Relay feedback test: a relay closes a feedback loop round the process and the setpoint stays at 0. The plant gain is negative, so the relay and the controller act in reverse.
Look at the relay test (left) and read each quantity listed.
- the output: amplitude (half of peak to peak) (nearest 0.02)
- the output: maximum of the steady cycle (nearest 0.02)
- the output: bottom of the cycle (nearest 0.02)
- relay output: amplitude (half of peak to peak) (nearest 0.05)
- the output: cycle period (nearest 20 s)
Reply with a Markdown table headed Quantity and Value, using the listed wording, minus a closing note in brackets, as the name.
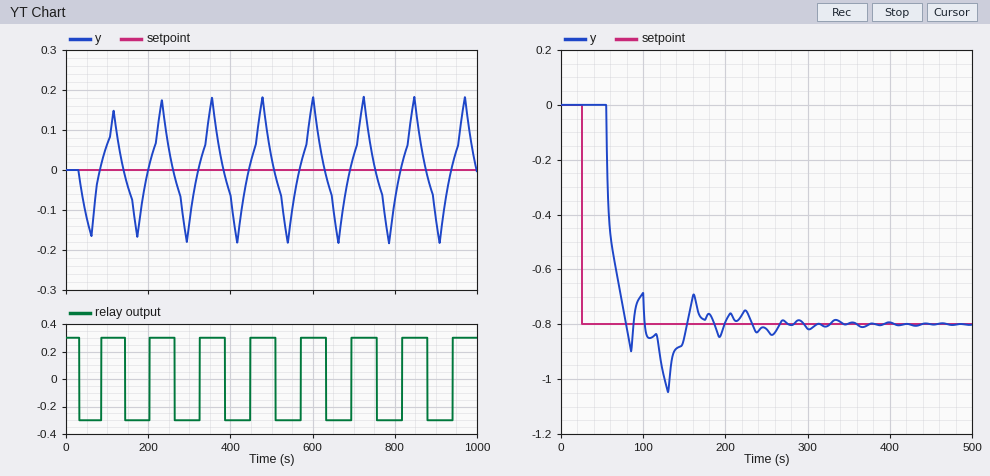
| Quantity | Value |
|---|---|
| the output: amplitude (half of peak to peak) | 0.18 |
| the output: maximum of the steady cycle | 0.18 |
| the output: bottom of the cycle | -0.18 |
| relay output: amplitude (half of peak to peak) | 0.30 |
| the output: cycle period | 120 s |
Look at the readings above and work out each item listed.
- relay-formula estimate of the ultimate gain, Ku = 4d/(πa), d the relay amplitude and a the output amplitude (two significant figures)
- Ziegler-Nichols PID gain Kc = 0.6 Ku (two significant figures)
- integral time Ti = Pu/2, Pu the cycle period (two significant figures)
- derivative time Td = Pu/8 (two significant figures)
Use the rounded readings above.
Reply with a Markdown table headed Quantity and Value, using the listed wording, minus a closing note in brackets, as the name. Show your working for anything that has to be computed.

| Quantity | Value |
|---|---|
| relay-formula estimate of the ultimate gain, Ku = 4d/(πa), d the relay amplitude and a the output amplitude | 4 × 0.3 / (π × 0.18) = 2.1 |
| Ziegler-Nichols PID gain Kc = 0.6 Ku | 0.6 × 2.1 = 1.3 |
| integral time Ti = Pu/2, Pu the cycle period | 120 / 2 = 60 s |
| derivative time Td = Pu/8 | 120 / 8 = 15 s |
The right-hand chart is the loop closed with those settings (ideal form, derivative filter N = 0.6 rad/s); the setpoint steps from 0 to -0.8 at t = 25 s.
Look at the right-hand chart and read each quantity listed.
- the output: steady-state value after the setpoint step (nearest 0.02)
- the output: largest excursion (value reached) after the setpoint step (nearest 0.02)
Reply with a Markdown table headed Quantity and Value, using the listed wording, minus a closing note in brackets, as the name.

| Quantity | Value |
|---|---|
| the output: steady-state value after the setpoint step | -0.80 |
| the output: largest excursion (value reached) after the setpoint step | -1.04 |
